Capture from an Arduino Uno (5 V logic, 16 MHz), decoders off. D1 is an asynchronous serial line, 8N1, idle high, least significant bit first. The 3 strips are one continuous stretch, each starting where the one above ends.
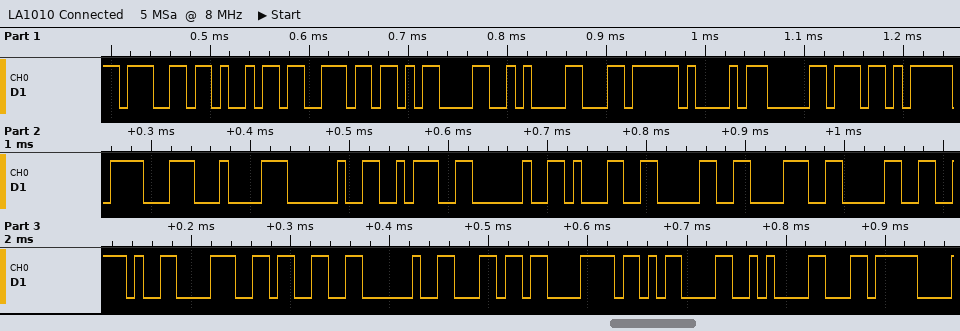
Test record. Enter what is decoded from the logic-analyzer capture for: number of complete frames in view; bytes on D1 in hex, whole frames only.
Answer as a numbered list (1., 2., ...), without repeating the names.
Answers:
1. 27
2. 67 69 6E 0D 0A EC A1 B0 EB 8F 84 20 3A 20 31 30 38 30 2E 38 33 20 6C 78 0D 0A EC
